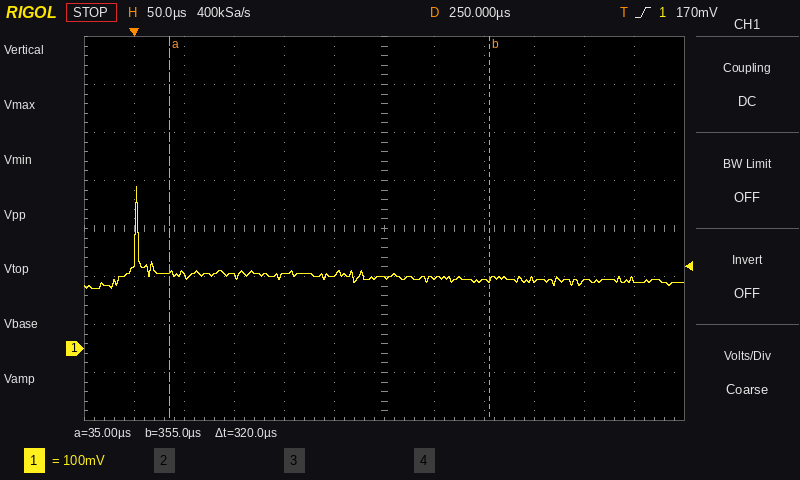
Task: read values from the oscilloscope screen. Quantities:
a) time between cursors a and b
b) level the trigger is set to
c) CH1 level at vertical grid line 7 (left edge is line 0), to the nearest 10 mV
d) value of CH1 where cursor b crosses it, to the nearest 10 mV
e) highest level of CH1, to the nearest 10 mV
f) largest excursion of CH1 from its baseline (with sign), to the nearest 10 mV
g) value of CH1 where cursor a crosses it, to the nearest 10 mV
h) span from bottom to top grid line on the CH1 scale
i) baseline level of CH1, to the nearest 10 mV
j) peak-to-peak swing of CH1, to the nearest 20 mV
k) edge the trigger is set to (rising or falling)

320 µs
170 mV
150 mV
140 mV
340 mV
+190 mV
160 mV
800 mV
150 mV
220 mV
rising
